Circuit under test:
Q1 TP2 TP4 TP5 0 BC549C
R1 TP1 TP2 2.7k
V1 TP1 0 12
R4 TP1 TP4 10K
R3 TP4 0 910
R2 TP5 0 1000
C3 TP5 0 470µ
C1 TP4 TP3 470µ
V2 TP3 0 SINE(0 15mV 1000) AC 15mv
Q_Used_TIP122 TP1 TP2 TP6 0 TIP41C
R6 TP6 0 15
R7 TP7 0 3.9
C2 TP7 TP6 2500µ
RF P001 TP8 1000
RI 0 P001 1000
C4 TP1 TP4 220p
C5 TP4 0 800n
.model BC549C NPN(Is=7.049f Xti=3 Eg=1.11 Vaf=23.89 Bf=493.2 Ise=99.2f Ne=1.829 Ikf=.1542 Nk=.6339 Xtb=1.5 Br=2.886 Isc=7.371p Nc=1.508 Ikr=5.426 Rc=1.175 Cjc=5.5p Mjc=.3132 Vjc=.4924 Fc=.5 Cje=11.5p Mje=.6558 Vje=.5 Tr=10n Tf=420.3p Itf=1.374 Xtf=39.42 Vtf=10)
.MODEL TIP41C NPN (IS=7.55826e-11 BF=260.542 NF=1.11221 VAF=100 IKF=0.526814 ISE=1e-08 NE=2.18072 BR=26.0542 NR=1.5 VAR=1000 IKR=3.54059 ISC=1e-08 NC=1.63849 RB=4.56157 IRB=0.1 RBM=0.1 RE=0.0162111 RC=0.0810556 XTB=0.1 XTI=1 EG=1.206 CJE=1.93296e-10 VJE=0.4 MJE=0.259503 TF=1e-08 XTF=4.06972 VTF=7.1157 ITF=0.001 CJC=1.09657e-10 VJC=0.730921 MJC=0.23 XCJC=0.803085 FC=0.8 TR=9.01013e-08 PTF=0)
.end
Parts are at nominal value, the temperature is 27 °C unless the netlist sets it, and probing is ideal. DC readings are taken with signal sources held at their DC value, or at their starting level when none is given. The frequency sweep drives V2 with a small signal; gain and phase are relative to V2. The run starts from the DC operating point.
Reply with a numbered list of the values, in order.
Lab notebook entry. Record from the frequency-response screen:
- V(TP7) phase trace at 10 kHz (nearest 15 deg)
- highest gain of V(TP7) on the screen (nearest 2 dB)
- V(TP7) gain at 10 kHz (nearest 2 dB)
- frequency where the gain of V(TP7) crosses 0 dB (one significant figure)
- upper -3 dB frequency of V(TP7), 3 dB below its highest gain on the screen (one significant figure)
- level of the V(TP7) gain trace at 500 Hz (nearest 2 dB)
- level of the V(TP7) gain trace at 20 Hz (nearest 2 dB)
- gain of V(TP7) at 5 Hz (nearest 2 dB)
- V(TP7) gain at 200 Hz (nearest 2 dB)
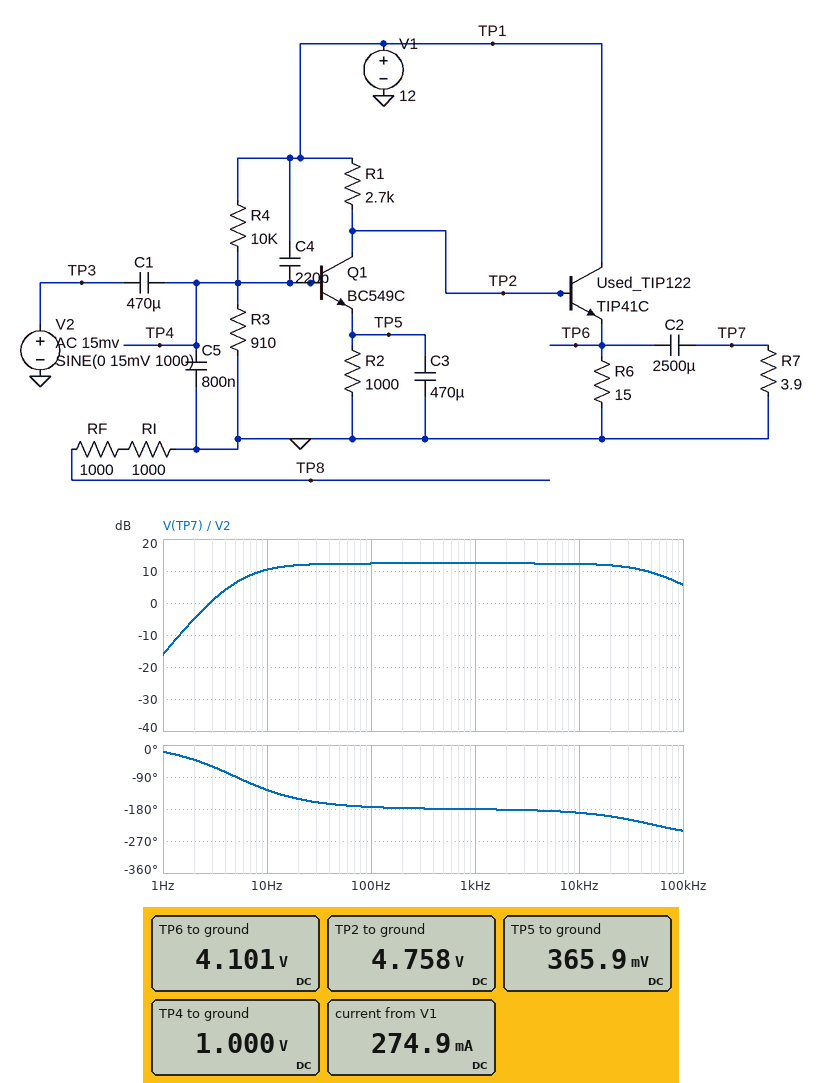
1. -195 deg
2. 12 dB
3. 12 dB
4. 3 Hz
5. 50 kHz
6. 12 dB
7. 12 dB
8. 6 dB
9. 12 dB
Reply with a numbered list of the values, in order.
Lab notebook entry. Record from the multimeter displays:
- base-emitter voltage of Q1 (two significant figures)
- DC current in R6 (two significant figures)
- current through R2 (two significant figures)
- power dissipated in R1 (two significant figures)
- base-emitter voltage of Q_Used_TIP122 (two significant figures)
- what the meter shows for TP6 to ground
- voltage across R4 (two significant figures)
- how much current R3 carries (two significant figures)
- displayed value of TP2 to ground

1. 630 mV
2. 270 mA
3. 370 µA
4. 19 mW
5. 660 mV
6. 4.101 V
7. 11 V
8. 1.1 mA
9. 4.758 V
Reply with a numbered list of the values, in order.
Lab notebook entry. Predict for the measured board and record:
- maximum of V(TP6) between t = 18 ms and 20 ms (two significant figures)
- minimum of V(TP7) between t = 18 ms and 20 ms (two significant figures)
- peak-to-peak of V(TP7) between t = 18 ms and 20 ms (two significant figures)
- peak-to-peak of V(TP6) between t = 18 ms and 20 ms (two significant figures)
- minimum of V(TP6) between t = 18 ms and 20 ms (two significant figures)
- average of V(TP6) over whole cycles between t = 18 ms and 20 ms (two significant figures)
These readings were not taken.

1. 4.1 V
2. -75 mV
3. 130 mV
4. 130 mV
5. 4.0 V
6. 4.1 V
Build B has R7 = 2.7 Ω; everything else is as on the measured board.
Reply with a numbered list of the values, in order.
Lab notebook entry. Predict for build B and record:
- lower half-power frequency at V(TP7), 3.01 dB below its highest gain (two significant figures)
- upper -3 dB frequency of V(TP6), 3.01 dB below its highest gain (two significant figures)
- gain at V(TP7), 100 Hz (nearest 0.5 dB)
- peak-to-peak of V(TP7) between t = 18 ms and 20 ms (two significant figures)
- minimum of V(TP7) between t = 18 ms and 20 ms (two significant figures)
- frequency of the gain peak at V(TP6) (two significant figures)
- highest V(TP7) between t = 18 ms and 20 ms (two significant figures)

1. 8.2 Hz
2. 16 Hz
3. 10.0 dB
4. 97 mV
5. -57 mV
6. 5.5 Hz
7. 40 mV
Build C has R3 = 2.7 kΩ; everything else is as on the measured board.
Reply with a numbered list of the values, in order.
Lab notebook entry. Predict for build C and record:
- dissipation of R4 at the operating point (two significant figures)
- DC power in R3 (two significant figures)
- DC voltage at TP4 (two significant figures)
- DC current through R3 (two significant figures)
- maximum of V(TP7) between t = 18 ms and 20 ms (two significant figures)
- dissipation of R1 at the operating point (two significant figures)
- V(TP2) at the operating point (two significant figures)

1. 8.9 mW
2. 2.4 mW
3. 2.5 V
4. 940 µA
5. 290 mV
6. 29 mW
7. 3.2 V
